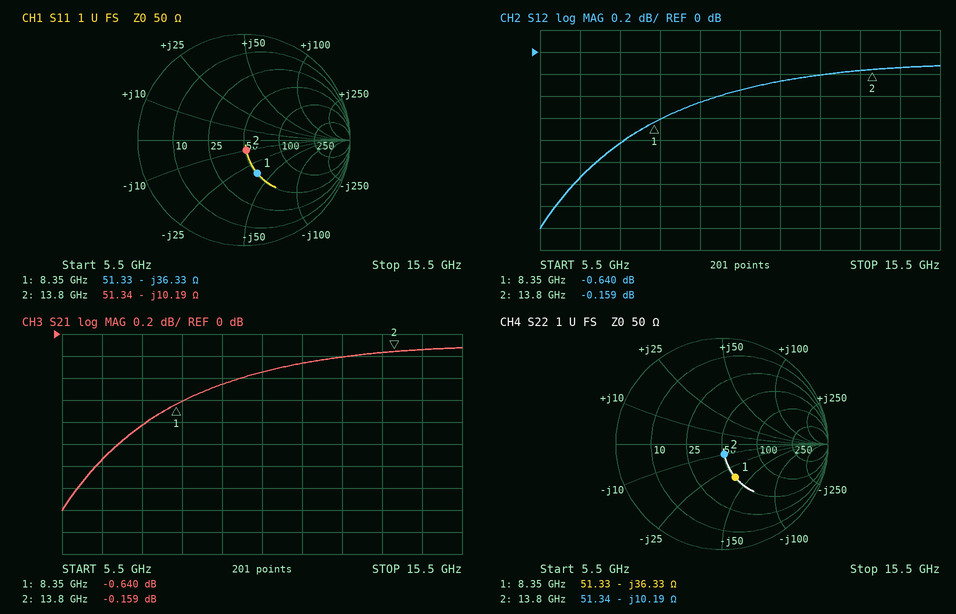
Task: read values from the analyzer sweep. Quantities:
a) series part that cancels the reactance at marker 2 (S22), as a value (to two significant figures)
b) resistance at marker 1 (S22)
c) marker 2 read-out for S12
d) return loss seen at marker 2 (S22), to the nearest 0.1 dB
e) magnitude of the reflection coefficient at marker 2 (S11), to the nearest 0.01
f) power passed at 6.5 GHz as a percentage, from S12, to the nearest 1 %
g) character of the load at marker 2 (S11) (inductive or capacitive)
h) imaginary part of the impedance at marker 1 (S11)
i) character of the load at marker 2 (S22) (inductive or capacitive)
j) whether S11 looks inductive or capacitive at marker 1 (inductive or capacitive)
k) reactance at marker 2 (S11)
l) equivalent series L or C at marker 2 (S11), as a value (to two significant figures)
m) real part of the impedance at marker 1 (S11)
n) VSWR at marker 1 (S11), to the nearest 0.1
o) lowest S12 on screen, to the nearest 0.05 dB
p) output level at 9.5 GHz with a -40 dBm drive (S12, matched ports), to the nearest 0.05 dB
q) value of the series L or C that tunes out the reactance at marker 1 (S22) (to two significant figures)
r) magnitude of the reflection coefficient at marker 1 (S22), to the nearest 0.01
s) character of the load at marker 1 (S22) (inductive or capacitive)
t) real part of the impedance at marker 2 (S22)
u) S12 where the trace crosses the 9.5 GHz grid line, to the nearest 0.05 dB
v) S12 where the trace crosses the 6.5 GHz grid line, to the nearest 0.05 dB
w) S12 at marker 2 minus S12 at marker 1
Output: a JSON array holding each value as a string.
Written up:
["120 pH", "51.33 Ω", "-0.159 dB", "19.9 dB", "0.10", "77 %", "capacitive", "-36.33 Ω", "capacitive", "capacitive", "-10.19 Ω", "1.1 pF", "51.33 Ω", "2.0", "-1.60 dB", "-40.45 dBm", "690 pH", "0.34", "capacitive", "51.34 Ω", "-0.45 dB", "-1.15 dB", "0.481 dB"]
